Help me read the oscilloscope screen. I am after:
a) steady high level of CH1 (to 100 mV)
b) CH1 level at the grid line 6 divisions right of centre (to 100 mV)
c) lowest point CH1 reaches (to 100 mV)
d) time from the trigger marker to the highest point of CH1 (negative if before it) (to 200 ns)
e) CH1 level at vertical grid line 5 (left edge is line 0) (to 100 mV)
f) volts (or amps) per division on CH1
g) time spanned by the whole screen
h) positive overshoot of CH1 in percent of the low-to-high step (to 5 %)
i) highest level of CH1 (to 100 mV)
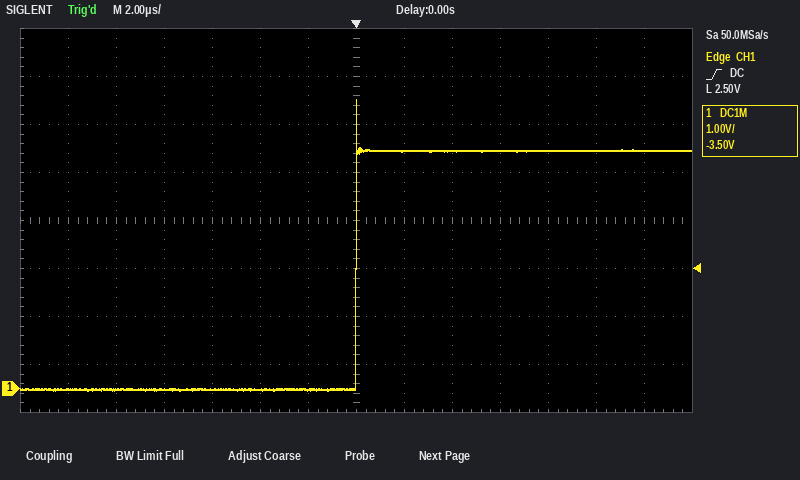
5.0 V
5.0 V
0.0 V
0.0 µs
0.0 V
1 V
28 µs
20 %
6.0 V
